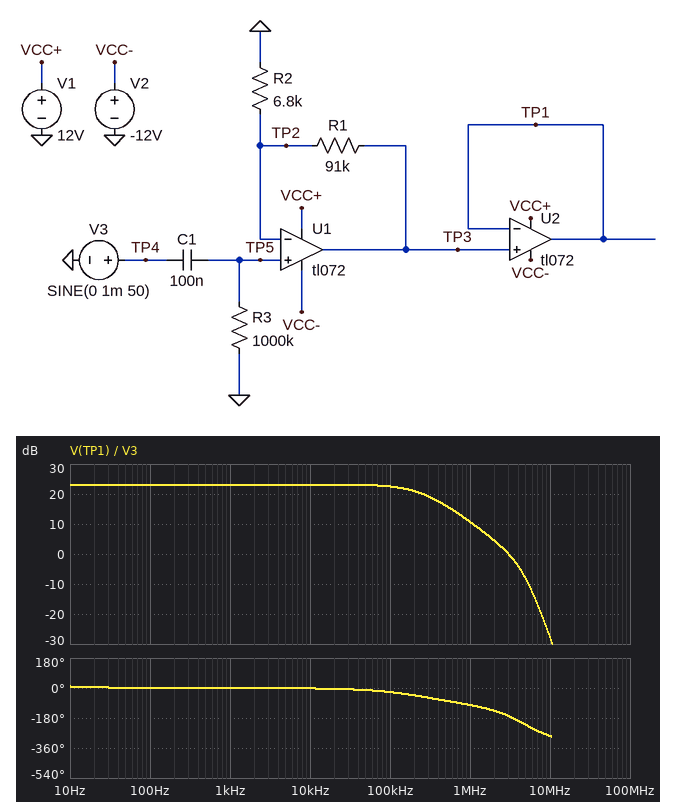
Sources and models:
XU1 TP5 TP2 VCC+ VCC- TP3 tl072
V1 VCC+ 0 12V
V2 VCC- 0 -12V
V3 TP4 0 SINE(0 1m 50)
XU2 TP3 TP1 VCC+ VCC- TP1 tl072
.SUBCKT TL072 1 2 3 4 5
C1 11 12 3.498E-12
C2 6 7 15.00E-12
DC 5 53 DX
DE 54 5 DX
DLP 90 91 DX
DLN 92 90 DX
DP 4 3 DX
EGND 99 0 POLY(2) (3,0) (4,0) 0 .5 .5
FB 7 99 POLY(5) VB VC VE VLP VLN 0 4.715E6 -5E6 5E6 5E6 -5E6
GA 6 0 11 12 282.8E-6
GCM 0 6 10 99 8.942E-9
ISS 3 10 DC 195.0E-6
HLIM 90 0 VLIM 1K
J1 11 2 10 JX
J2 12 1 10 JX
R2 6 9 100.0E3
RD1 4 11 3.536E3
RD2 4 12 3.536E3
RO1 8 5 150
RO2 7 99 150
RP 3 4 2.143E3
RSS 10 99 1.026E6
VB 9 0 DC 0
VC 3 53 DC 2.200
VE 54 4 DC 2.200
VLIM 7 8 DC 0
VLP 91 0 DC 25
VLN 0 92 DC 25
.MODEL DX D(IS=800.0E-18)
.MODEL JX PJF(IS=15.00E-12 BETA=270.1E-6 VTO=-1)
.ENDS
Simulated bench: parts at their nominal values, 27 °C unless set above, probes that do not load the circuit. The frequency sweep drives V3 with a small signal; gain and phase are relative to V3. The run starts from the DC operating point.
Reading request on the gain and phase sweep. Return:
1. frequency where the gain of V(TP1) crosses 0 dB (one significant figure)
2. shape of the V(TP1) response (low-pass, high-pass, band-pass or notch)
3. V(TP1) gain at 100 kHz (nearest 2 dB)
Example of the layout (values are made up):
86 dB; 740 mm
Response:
3 MHz; low-pass; 22 dB
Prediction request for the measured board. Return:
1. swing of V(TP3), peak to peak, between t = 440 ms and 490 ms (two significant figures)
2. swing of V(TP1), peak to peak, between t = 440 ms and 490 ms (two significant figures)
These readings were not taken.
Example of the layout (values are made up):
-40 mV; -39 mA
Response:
29 mV; 29 mV
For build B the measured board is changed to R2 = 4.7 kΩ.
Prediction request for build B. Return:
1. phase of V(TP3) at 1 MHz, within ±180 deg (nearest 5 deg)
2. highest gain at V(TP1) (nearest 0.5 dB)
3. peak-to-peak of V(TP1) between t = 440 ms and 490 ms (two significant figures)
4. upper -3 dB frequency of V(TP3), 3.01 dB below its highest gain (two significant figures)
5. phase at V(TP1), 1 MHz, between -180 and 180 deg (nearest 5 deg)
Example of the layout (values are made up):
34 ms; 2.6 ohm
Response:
-90 deg; 26.0 dB; 41 mV; 170 kHz; -105 deg
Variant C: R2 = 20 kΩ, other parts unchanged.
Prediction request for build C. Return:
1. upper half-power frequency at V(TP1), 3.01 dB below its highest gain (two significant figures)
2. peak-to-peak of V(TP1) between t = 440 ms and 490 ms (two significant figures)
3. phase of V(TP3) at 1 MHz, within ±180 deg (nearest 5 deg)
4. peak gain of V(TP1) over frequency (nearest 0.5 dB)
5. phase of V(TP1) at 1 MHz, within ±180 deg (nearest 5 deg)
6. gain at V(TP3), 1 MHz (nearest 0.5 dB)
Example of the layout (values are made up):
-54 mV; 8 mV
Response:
690 kHz; 11 mV; -65 deg; 15.0 dB; -80 deg; 10.0 dB
